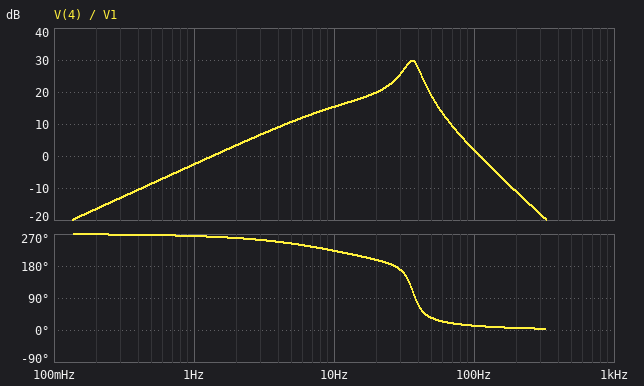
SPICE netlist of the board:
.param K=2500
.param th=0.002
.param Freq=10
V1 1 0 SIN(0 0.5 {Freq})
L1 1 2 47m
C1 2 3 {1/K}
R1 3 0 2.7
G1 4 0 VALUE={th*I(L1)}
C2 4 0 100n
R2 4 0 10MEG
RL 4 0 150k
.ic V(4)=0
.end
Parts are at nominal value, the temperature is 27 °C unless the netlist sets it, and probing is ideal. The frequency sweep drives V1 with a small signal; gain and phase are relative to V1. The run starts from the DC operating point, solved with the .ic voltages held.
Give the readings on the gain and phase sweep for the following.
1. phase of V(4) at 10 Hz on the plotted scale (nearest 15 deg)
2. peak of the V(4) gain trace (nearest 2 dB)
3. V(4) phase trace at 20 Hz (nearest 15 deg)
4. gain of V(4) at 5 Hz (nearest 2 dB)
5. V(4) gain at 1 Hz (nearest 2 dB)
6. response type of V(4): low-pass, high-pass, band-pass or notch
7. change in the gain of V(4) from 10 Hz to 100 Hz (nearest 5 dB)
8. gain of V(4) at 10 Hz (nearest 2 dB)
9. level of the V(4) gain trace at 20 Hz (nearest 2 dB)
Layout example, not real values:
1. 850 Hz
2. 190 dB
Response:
1. 225 deg
2. 30 dB
3. 195 deg
4. 10 dB
5. -2 dB
6. band-pass
7. -15 dB
8. 16 dB
9. 20 dB
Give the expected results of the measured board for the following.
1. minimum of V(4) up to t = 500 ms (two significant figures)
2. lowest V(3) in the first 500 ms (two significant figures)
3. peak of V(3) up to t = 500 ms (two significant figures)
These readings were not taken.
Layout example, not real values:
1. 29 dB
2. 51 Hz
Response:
1. -2.9 V
2. -43 mV
3. 51 mV
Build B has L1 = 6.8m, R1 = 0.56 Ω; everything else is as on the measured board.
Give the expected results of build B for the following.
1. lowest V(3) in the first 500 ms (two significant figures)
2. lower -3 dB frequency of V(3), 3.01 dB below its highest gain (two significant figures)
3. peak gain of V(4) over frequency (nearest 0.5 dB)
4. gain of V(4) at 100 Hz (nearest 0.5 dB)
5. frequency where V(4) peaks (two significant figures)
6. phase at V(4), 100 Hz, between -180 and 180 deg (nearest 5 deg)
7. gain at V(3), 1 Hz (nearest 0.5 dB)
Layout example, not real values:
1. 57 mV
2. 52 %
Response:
1. -7.9 mV
2. 90 Hz
3. 35.5 dB
4. 34.0 dB
5. 96 Hz
6. 70 deg
7. -57.0 dB
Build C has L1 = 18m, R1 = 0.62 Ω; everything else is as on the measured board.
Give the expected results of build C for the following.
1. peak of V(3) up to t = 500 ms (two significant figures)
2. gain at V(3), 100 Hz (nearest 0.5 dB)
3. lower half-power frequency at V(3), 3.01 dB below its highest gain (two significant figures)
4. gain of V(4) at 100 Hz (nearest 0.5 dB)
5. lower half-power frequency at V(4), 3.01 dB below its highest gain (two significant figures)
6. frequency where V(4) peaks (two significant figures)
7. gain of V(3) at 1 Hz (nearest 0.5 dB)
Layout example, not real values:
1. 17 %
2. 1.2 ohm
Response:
1. 14 mV
2. -21.5 dB
3. 57 Hz
4. 12.5 dB
5. 56 Hz
6. 59 Hz
7. -56.0 dB
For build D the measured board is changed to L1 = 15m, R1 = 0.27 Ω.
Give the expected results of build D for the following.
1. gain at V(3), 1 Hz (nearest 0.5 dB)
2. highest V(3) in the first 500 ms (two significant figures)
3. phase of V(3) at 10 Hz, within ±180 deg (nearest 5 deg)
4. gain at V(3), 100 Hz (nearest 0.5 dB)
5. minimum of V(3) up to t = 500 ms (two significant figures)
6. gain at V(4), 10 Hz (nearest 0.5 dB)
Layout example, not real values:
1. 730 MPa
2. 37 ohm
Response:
1. -63.5 dB
2. 6.3 mV
3. 90 deg
4. -26.0 dB
5. -5.7 mV
6. 15.0 dB
